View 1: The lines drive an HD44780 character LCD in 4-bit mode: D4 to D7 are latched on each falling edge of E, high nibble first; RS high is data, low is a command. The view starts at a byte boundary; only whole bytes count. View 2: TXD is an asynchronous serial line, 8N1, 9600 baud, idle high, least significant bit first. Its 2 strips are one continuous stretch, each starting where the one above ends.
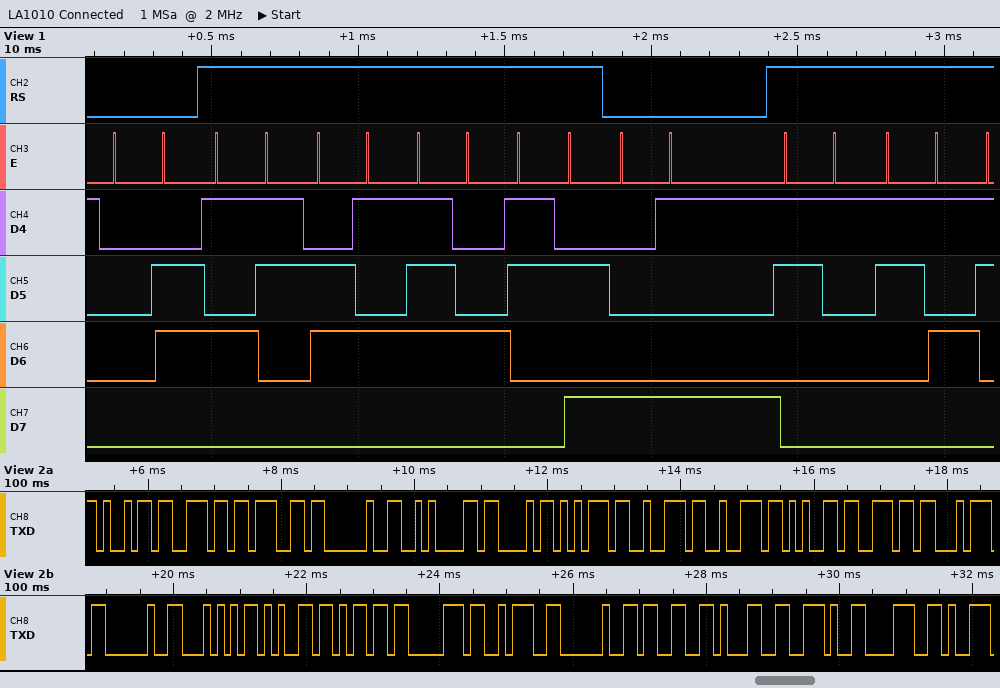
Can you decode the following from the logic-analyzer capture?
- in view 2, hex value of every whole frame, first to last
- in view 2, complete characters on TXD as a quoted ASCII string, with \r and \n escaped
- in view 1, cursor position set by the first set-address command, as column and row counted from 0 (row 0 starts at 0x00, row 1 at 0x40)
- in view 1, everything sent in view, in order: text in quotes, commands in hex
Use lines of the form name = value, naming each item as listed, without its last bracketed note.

in view 2, hex value of every whole frame, first to last = 69 6E 67 20 0A 43 75 72 72 65 6E 74 20 54 65 6D 70 3A 20 33 31 2E 38
in view 2, complete characters on TXD as a quoted ASCII string, with \r and \n escaped = "ing \nCurrent Temp: 31.8"
in view 1, cursor position set by the first set-address command, as column and row counted from 0 = column 9, row 0
in view 1, everything sent in view, in order: text in quotes, commands in hex = 0x06 "Set:" 0x89 "15"
